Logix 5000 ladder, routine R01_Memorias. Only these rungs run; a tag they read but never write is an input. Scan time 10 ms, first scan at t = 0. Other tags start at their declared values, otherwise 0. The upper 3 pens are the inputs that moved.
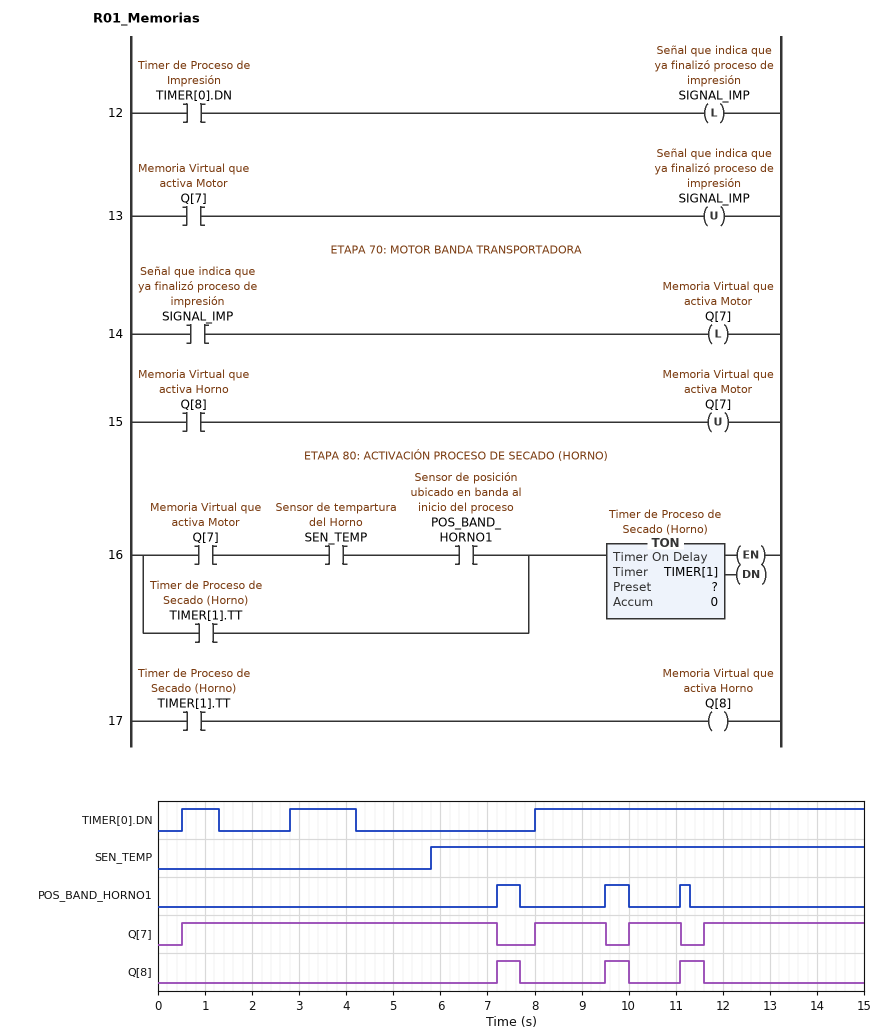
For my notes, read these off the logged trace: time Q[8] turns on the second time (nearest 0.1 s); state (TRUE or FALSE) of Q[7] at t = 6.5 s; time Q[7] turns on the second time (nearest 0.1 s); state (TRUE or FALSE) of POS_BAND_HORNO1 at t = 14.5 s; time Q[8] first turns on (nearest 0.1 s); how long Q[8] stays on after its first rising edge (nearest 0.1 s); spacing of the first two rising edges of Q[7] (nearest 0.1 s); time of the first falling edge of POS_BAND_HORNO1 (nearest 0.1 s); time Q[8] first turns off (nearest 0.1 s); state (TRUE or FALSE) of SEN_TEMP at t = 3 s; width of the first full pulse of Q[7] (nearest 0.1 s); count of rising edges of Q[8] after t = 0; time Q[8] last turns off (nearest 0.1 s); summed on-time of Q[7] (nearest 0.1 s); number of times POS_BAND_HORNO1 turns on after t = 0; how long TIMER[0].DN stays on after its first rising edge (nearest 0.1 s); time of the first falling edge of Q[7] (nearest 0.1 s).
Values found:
9.5 s
TRUE
8.0 s
FALSE
7.2 s
0.5 s
7.5 s
7.7 s
7.7 s
FALSE
6.7 s
3
11.6 s
12.7 s
3
0.8 s
7.2 s
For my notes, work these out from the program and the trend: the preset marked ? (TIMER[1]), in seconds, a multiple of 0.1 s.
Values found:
0.5 s
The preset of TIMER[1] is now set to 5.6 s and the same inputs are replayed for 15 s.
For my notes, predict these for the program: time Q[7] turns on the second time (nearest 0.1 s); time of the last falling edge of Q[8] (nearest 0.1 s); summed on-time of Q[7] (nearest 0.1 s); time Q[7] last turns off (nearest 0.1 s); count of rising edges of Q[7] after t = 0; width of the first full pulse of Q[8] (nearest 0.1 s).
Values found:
12.8 s
12.8 s
8.9 s
7.2 s
2
5.6 s
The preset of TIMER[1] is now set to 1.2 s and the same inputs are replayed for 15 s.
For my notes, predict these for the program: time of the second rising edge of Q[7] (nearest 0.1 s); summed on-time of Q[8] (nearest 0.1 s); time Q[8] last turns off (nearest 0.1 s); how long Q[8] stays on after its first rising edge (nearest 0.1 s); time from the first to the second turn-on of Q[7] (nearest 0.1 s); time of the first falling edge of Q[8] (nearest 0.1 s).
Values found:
8.4 s
3.6 s
12.3 s
1.2 s
7.9 s
8.4 s
